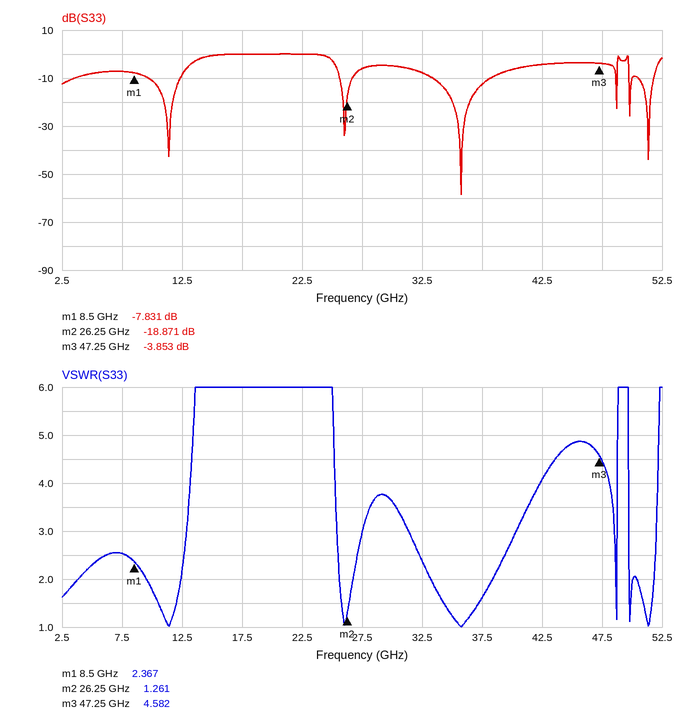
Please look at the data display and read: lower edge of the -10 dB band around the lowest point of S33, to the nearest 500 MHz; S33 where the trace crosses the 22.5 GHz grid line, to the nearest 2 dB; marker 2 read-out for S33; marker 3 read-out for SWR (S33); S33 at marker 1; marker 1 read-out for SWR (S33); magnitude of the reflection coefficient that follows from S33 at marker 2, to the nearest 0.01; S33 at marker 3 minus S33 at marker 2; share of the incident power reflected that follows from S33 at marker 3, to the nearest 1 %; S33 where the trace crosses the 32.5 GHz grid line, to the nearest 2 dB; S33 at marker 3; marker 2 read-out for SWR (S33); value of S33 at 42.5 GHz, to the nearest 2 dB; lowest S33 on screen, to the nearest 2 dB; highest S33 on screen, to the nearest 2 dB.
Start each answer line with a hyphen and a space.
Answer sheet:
- 33.5 GHz
- 0 dB
- -18.871 dB
- 4.582
- -7.831 dB
- 2.367
- 0.11
- 15.018 dB
- 41 %
- -8 dB
- -3.853 dB
- 1.261
- -4 dB
- -58 dB
- 0 dB
